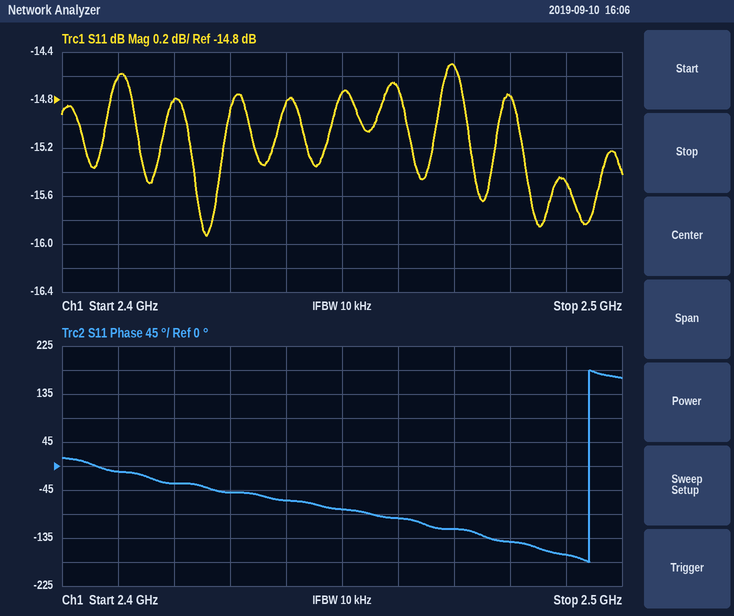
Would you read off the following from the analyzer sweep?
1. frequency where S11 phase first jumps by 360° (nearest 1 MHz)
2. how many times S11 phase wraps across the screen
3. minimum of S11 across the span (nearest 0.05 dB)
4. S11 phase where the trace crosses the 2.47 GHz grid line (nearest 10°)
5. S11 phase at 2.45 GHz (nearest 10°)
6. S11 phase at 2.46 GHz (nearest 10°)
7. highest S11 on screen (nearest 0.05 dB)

2.494 GHz
1
-15.95 dB
-120°
-80°
-100°
-14.50 dB
